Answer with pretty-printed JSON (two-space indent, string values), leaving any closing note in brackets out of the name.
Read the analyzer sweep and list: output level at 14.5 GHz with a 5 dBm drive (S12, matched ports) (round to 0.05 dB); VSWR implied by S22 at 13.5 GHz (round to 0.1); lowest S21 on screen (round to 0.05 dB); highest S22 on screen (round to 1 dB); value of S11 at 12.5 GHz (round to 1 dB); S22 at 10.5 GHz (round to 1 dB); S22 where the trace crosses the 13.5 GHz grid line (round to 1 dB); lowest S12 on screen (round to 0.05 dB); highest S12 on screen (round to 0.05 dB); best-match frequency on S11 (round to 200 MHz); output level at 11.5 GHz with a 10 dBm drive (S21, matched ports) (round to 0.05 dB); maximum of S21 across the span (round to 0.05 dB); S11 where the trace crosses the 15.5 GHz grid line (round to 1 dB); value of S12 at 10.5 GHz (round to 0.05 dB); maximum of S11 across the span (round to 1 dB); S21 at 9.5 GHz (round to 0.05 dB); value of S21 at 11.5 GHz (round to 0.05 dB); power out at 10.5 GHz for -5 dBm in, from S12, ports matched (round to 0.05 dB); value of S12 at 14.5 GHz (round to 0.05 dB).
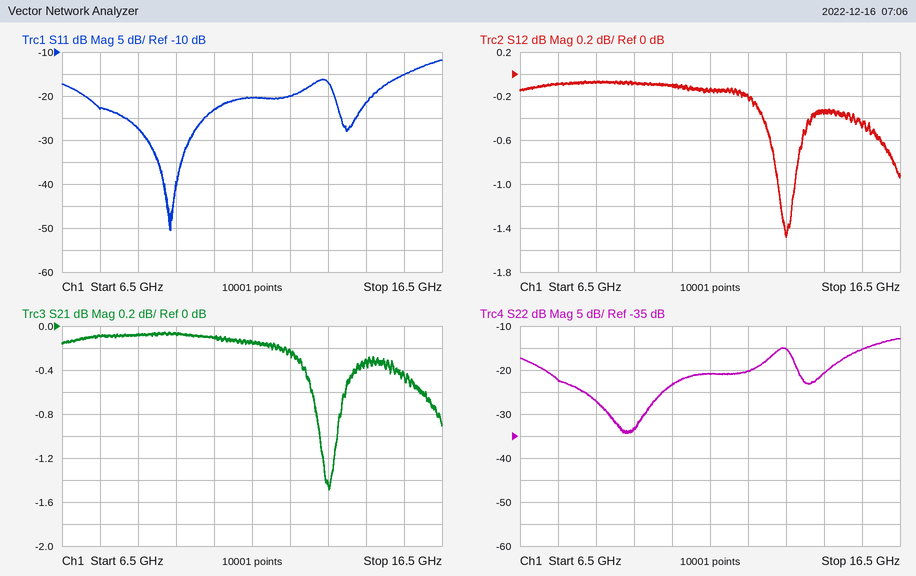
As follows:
{
  "output level at 14.5 GHz with a 5 dBm drive (S12, matched ports)": "4.65 dBm",
  "VSWR implied by S22 at 13.5 GHz": "1.4",
  "lowest S21 on screen": "-1.50 dB",
  "highest S22 on screen": "-13 dB",
  "value of S11 at 12.5 GHz": "-20 dB",
  "S22 at 10.5 GHz": "-23 dB",
  "S22 where the trace crosses the 13.5 GHz grid line": "-15 dB",
  "lowest S12 on screen": "-1.50 dB",
  "highest S12 on screen": "-0.05 dB",
  "best-match frequency on S11": "9.4 GHz",
  "output level at 11.5 GHz with a 10 dBm drive (S21, matched ports)": "9.85 dBm",
  "maximum of S21 across the span": "-0.05 dB",
  "S11 where the trace crosses the 15.5 GHz grid line": "-15 dB",
  "value of S12 at 10.5 GHz": "-0.10 dB",
  "maximum of S11 across the span": "-12 dB",
  "S21 at 9.5 GHz": "-0.05 dB",
  "value of S21 at 11.5 GHz": "-0.15 dB",
  "power out at 10.5 GHz for -5 dBm in, from S12, ports matched": "-5.10 dBm",
  "value of S12 at 14.5 GHz": "-0.35 dB"
}
